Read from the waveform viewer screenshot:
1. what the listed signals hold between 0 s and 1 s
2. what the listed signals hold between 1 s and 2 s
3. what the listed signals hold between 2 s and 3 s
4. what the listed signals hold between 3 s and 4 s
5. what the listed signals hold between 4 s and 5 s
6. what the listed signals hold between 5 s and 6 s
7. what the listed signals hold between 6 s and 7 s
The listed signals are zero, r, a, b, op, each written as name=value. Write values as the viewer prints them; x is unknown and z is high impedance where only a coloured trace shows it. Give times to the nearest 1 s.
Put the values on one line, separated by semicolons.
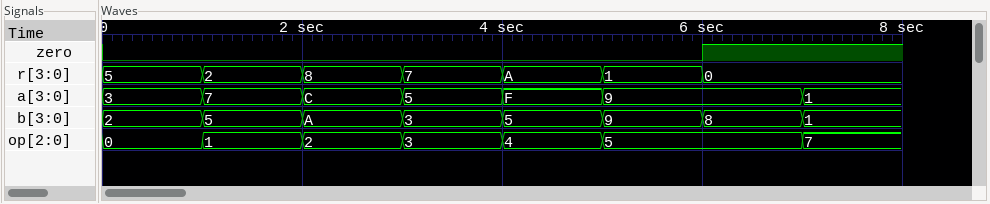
zero=0, r=5, a=3, b=2, op=0; zero=0, r=2, a=7, b=5, op=1; zero=0, r=8, a=C, b=A, op=2; zero=0, r=7, a=5, b=3, op=3; zero=0, r=A, a=F, b=5, op=4; zero=0, r=1, a=9, b=9, op=5; zero=1, r=0, a=9, b=8, op=5
